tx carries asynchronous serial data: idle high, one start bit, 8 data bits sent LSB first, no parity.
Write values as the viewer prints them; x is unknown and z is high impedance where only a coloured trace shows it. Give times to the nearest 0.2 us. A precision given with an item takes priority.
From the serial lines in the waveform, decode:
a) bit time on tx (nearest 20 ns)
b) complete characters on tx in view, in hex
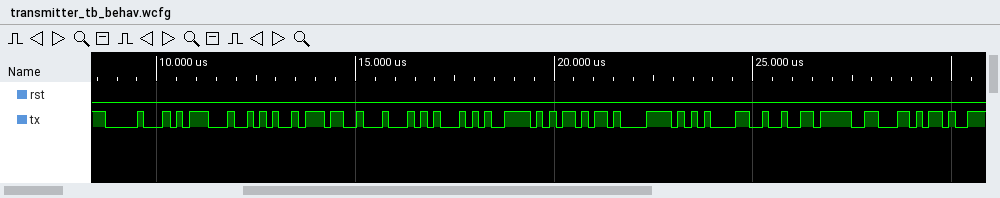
160 ns
10, 1D, 2A, 37, 44, 51, 5E, 6B, 78, 85, 92, 9F, AC
